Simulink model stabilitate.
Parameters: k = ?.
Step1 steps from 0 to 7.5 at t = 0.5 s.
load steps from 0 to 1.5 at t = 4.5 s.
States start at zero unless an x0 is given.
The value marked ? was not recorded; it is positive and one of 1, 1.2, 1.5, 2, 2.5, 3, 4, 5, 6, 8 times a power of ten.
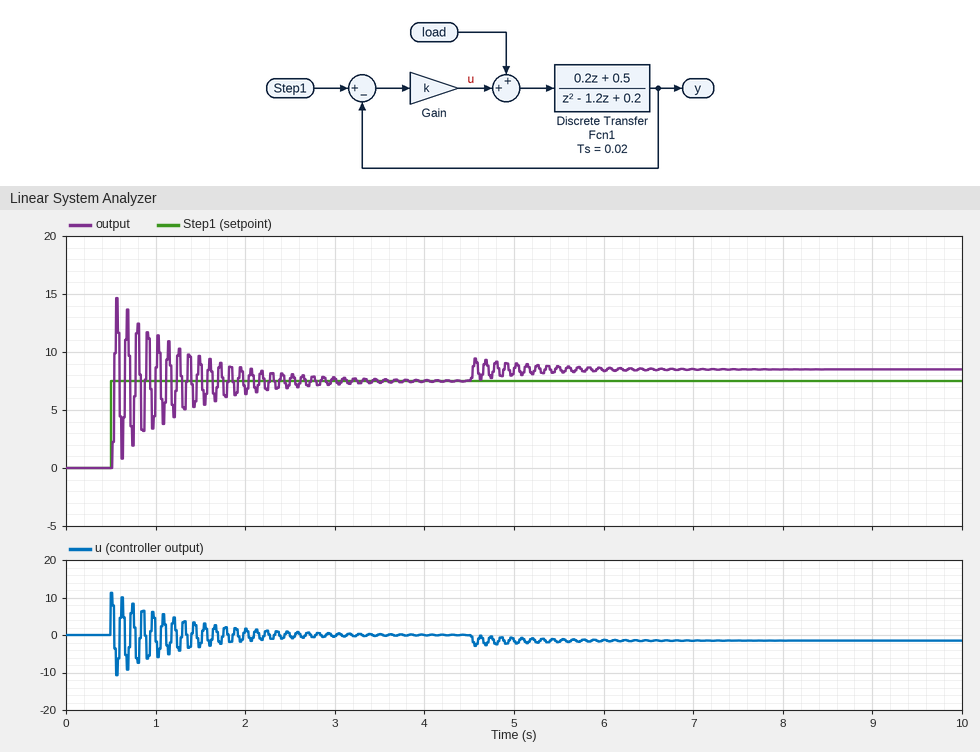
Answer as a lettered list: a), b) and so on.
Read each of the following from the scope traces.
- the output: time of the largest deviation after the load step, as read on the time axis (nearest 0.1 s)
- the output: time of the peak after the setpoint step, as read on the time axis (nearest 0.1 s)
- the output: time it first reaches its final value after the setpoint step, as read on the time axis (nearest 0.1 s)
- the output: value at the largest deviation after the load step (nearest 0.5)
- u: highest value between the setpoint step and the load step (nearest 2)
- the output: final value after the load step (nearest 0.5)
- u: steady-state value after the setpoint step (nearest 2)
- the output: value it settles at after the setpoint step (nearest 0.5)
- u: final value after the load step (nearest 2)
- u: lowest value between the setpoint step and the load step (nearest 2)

a) 4.6 s
b) 0.6 s
c) 0.5 s
d) 9.5
e) 12
f) 8.5
g) 0
h) 7.5
i) -2
j) -10
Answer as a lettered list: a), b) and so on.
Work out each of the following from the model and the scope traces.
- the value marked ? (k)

a) 1.5
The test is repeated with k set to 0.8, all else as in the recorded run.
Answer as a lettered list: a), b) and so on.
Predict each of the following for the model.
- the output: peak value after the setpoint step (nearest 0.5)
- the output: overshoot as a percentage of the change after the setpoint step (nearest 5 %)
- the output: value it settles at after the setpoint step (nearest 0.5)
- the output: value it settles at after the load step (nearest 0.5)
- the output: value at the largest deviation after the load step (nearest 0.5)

a) 10.5
b) 40 %
c) 7.5
d) 9.5
e) 10.0
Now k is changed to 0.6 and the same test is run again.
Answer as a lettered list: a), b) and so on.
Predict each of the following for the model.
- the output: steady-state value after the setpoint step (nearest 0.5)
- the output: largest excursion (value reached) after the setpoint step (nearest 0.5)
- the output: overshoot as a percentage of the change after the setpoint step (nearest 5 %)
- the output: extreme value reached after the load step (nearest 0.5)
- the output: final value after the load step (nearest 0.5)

a) 7.5
b) 9.0
c) 20 %
d) 10.5
e) 10.0
